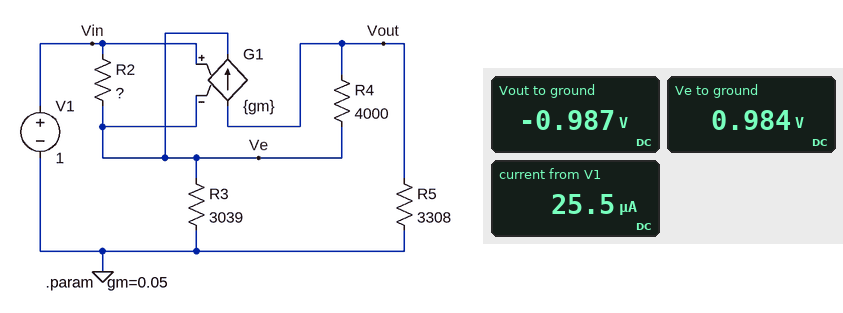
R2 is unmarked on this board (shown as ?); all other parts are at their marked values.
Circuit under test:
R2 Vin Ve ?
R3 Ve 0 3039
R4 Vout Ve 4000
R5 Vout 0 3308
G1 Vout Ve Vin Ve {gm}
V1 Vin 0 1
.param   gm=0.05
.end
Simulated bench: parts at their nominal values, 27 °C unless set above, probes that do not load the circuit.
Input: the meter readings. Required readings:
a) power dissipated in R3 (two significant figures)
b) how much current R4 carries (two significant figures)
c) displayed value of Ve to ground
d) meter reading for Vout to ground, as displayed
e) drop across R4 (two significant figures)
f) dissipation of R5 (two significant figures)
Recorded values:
320 µW
490 µA
0.984 V
-0.987 V
2.0 V
290 µW
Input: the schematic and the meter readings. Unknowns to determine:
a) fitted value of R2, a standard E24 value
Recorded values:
620 Ω
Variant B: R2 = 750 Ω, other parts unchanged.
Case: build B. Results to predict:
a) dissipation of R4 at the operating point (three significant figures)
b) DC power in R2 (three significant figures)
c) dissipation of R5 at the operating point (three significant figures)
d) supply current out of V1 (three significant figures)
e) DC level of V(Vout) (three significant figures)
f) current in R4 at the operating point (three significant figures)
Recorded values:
985 µW
340 nW
303 µW
21.3 µA
-1.00 V
496 µA
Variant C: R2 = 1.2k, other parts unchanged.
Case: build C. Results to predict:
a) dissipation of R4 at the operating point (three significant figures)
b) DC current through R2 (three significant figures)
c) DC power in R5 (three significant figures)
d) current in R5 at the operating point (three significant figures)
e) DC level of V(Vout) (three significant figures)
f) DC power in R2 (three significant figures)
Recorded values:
1.01 mW
13.5 µA
318 µW
310 µA
-1.03 V
220 nW
